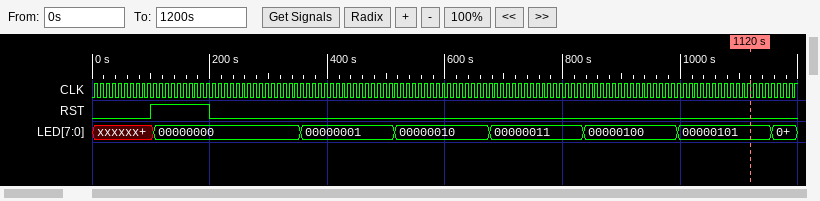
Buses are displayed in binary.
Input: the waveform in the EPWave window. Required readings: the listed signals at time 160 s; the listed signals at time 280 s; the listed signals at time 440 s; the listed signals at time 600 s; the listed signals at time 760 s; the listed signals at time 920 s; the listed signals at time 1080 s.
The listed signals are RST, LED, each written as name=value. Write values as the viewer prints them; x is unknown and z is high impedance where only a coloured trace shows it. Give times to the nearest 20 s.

RST=1, LED=00000000
RST=0, LED=00000000
RST=0, LED=00000001
RST=0, LED=00000010
RST=0, LED=00000011
RST=0, LED=00000100
RST=0, LED=00000101
